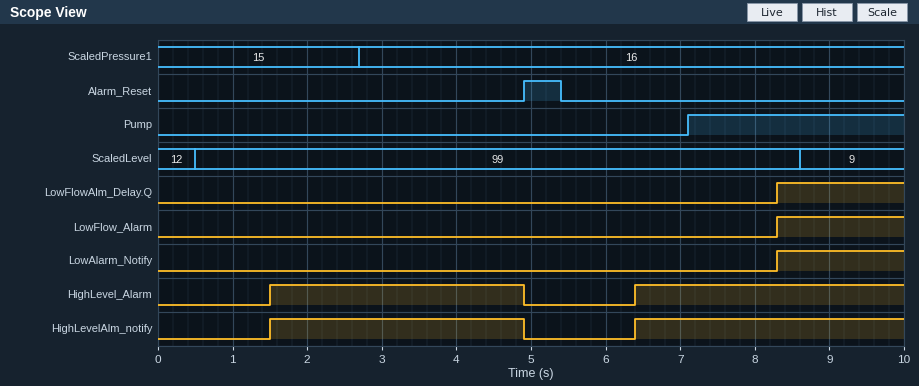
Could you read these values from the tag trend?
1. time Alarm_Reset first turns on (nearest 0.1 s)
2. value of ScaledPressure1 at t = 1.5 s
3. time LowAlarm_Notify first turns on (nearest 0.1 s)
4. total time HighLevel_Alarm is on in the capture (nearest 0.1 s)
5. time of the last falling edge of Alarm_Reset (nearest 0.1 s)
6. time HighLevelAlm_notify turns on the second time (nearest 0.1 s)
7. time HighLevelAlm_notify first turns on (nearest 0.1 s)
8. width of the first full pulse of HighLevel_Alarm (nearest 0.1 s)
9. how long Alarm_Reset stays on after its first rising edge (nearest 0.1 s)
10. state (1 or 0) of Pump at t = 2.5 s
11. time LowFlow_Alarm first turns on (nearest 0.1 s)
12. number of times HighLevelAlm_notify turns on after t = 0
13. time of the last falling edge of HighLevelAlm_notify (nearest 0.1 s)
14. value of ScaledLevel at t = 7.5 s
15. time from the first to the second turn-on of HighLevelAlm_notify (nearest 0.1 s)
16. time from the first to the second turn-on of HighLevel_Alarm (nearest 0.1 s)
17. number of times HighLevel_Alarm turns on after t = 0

4.9 s
15
8.3 s
7.0 s
5.4 s
6.4 s
1.5 s
3.4 s
0.5 s
0
8.3 s
2
4.9 s
99
4.9 s
4.9 s
2
